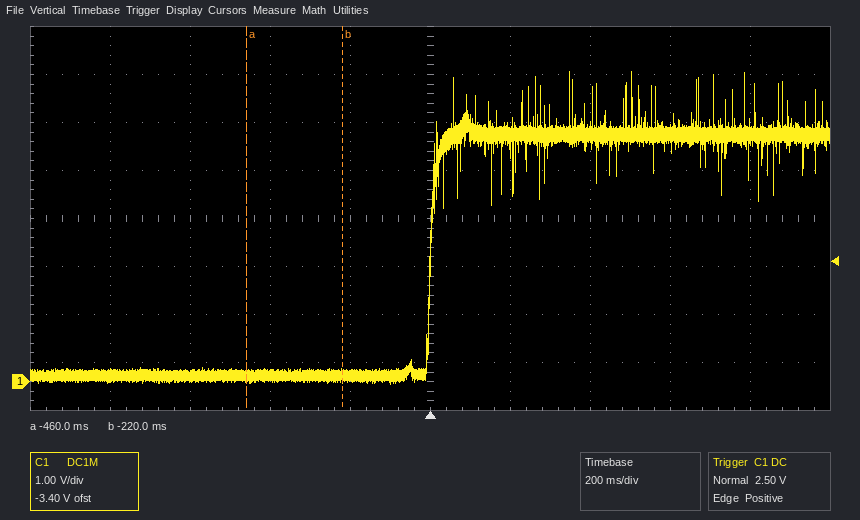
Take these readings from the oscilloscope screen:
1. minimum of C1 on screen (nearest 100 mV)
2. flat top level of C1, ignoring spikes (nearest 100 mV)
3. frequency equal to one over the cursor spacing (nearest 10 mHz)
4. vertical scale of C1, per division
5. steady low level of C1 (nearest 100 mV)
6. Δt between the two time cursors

0.0 V
5.2 V
4.17 Hz
1 V
100 mV
240 ms
